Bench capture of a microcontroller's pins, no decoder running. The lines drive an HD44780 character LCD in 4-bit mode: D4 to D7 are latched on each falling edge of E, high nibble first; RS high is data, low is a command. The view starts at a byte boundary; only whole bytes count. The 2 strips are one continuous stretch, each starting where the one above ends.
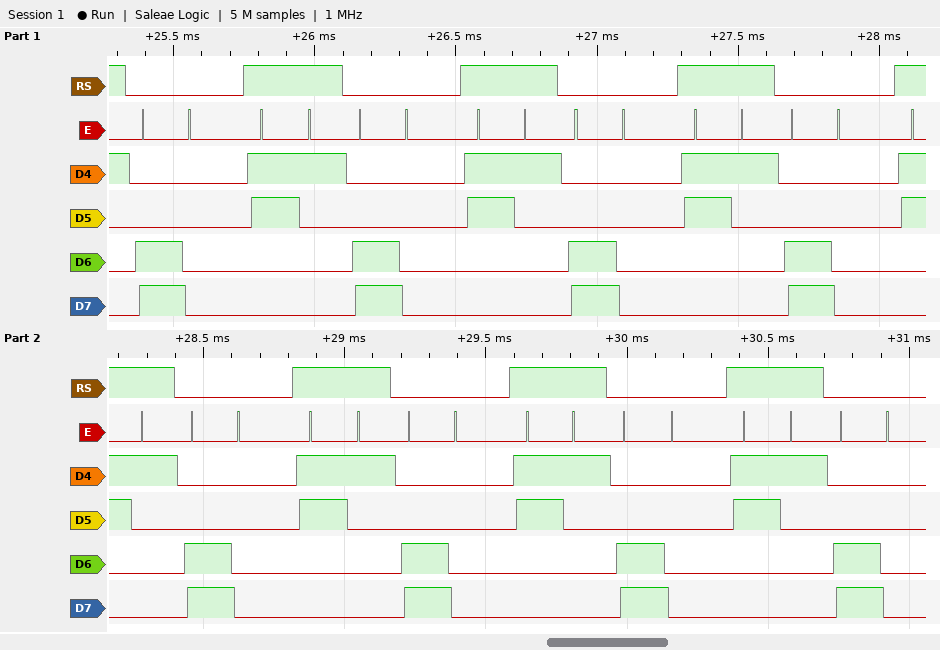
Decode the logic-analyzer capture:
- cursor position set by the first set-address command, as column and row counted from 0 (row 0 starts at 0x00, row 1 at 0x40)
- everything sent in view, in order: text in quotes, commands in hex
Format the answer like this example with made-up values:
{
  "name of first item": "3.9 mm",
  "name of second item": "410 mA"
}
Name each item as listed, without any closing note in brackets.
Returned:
{
  "cursor position set by the first set-address command, as column and row counted from 0": "column 0, row 1",
  "everything sent in view, in order: text in quotes, commands in hex": "0xC0 \"1\" 0xC0 \"1\" 0xC0 \"1\" 0xC0 \"1\" 0xC0 \"1\" 0xC0 \"1\" 0xC0 \"1\" 0xC0"
}
